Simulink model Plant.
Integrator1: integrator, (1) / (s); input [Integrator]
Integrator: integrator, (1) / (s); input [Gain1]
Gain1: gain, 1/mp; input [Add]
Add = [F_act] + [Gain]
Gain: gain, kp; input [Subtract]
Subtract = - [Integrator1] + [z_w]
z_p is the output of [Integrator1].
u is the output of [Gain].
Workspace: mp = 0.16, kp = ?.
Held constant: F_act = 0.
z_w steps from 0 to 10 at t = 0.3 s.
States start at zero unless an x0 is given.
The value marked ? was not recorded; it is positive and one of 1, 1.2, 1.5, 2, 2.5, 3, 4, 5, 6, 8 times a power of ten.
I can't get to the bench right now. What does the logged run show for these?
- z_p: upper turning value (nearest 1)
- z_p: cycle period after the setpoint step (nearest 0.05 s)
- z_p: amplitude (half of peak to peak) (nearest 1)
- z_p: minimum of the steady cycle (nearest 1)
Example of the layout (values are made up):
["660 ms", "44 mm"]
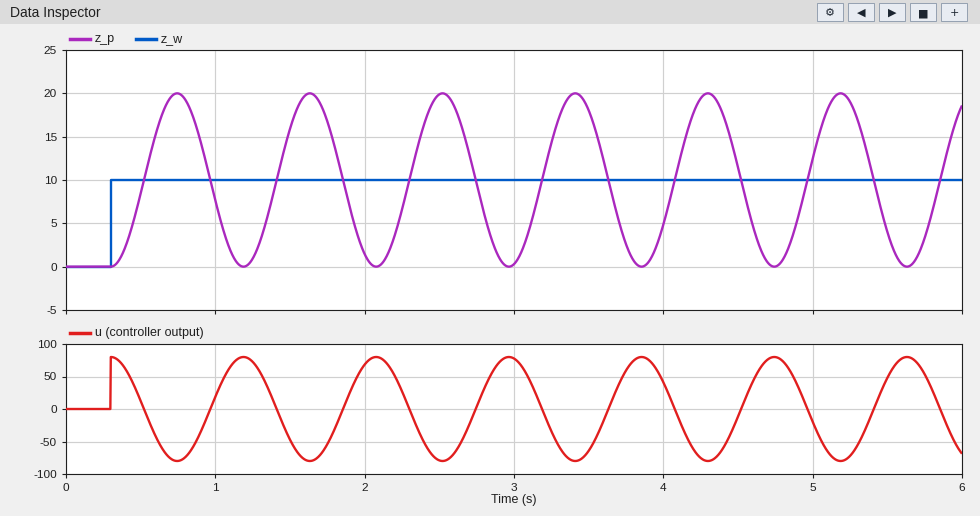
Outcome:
["20", "0.90 s", "10", "0"]
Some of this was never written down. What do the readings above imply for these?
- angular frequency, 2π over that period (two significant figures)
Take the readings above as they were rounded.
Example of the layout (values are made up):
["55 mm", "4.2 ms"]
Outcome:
["7.0 rad/s"]
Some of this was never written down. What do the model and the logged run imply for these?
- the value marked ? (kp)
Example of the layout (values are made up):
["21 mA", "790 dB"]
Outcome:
["8"]
